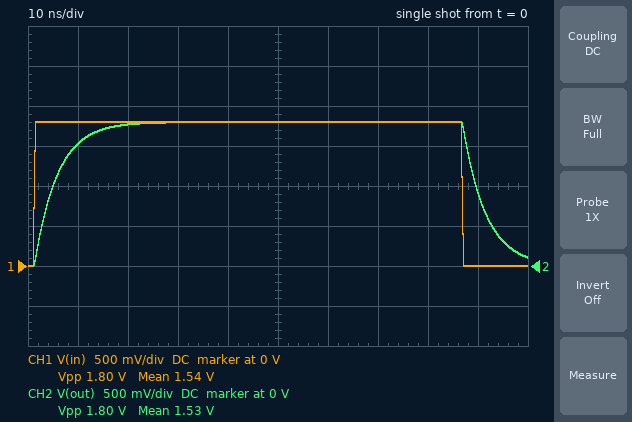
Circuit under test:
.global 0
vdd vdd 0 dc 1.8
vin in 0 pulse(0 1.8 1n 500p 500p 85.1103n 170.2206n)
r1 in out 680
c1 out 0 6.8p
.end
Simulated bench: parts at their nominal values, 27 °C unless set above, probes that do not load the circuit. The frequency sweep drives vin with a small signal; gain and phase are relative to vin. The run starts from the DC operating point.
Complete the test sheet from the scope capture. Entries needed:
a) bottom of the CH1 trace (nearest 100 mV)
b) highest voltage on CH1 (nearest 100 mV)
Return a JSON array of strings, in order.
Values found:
["0 V", "1.8 V"]
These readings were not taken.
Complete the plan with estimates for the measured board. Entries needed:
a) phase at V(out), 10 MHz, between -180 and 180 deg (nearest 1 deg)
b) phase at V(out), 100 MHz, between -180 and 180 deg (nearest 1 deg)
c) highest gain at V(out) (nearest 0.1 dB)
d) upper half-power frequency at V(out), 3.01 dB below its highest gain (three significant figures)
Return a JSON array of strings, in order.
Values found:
["-16 deg", "-71 deg", "0 dB", "34.4 MHz"]
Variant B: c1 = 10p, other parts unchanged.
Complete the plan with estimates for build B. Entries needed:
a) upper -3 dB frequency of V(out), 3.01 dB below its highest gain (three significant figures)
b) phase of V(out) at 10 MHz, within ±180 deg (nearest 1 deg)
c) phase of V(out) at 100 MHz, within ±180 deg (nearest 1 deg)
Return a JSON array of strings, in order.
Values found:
["23.4 MHz", "-23 deg", "-77 deg"]
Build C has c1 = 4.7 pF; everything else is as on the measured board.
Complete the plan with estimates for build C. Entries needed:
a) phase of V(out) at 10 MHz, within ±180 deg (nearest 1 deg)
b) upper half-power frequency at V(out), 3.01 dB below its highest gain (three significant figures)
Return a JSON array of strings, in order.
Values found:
["-11 deg", "49.8 MHz"]
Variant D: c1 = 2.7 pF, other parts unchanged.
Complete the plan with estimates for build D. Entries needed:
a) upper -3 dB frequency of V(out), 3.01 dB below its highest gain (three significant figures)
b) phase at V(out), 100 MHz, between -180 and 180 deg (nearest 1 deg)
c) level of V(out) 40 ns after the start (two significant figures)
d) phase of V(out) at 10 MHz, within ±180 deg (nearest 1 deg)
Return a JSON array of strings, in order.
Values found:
["86.7 MHz", "-49 deg", "1.8 V", "-7 deg"]
